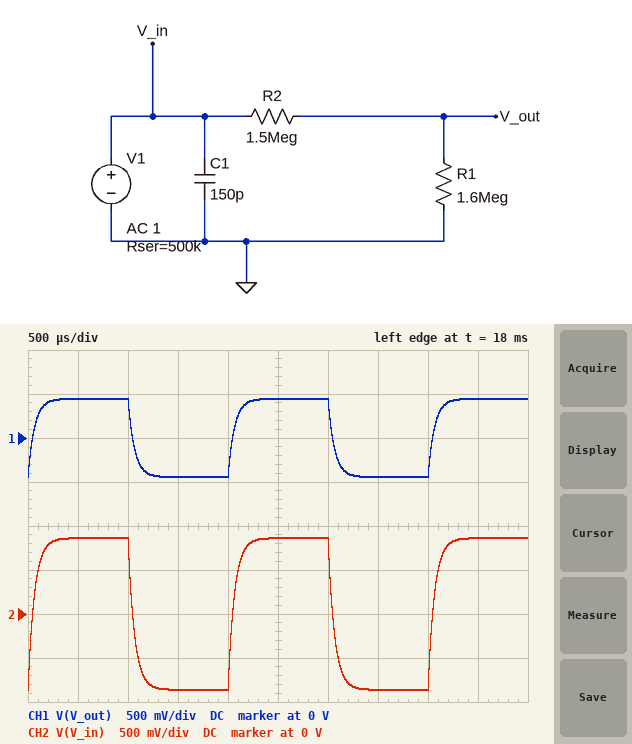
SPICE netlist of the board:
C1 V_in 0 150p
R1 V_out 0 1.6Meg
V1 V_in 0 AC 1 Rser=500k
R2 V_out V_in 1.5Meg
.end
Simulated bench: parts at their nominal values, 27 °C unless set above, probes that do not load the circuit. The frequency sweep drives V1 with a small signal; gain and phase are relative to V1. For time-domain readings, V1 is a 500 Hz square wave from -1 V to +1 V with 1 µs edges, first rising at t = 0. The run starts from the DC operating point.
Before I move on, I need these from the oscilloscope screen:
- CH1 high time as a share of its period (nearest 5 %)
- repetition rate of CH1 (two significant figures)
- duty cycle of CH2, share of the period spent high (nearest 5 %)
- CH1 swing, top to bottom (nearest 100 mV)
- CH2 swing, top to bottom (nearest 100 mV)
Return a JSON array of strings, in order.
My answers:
["50 %", "500 Hz", "50 %", "900 mV", "1.7 V"]
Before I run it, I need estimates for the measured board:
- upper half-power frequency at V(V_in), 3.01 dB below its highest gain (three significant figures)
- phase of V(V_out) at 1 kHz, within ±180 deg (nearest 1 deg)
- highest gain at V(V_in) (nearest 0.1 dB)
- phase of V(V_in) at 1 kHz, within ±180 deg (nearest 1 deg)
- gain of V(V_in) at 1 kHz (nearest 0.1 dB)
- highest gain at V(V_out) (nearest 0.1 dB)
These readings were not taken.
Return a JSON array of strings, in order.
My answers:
["2.46 kHz", "-22 deg", "-1.3 dB", "-22 deg", "-2.0 dB", "-7.0 dB"]
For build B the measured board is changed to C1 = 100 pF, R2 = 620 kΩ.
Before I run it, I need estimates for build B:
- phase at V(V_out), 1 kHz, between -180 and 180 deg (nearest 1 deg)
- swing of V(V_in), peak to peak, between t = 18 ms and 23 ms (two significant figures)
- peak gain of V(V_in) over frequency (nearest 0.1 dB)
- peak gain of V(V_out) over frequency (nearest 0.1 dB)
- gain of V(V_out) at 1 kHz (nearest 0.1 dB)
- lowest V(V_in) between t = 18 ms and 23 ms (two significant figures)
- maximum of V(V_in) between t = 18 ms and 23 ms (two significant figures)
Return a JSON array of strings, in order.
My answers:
["-14 deg", "1.6 V", "-1.8 dB", "-4.6 dB", "-4.9 dB", "-820 mV", "820 mV"]
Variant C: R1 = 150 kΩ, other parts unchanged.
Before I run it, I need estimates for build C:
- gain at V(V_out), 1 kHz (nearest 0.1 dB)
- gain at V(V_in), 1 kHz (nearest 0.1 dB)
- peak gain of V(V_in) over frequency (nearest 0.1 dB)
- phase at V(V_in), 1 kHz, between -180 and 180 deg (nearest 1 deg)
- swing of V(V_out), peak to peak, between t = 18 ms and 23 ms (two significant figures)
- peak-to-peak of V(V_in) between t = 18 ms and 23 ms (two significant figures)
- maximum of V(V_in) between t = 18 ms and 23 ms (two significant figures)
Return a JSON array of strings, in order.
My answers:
["-23.7 dB", "-2.8 dB", "-2.3 dB", "-20 deg", "140 mV", "1.5 V", "770 mV"]
